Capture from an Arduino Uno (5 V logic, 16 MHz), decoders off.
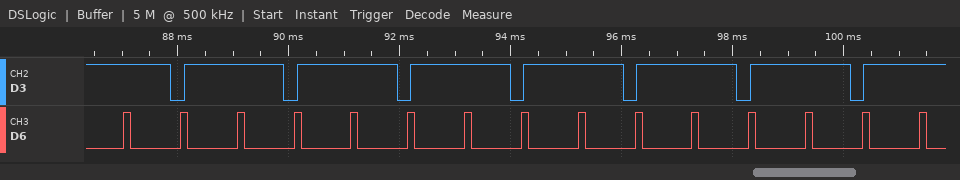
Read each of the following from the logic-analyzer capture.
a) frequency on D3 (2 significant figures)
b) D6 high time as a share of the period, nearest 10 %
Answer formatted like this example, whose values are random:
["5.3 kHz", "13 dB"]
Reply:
["490 Hz", "10 %"]
